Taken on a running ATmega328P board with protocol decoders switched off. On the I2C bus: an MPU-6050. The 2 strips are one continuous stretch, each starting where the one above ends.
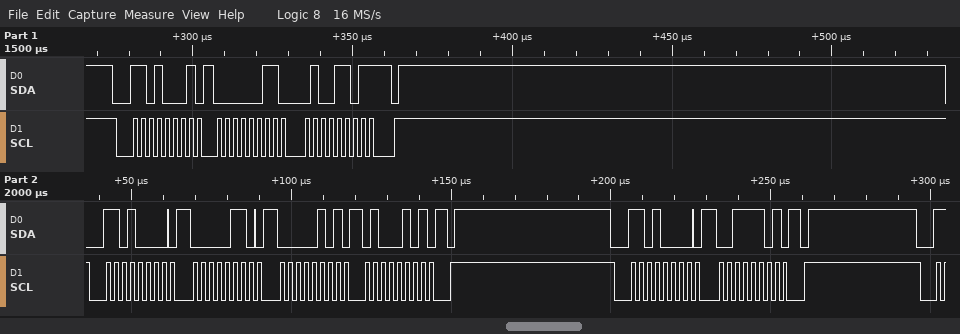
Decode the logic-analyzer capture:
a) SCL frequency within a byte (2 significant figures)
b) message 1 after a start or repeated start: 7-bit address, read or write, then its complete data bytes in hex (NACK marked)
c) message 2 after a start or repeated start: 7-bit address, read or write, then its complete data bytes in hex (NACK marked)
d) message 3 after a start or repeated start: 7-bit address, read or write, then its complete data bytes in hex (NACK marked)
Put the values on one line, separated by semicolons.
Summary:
400 kHz; 0x68 read: 03 4D NACK; 0x68 write: 06 05 45; 0x68 write: 3D
